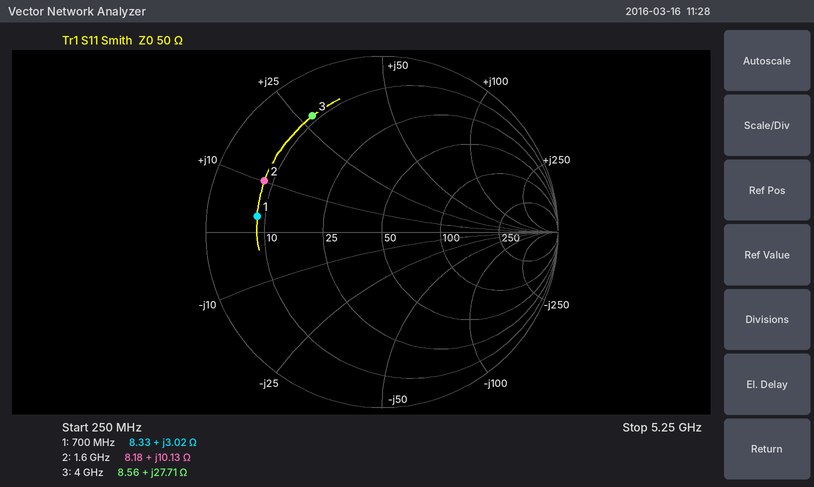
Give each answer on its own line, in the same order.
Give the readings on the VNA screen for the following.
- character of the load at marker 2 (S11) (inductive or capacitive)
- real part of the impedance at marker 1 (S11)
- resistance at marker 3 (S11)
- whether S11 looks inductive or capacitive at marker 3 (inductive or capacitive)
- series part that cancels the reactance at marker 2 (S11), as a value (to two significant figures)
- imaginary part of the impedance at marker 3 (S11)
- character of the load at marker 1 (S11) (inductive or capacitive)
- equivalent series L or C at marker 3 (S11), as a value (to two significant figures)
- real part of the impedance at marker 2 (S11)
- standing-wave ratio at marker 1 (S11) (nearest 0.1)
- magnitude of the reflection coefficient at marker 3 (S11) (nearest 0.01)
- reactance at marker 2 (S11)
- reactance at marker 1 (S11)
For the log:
inductive
8.33 Ω
8.56 Ω
inductive
9.8 pF
+27.71 Ω
inductive
1.1 nH
8.18 Ω
6.0
0.77
+10.13 Ω
+3.02 Ω
